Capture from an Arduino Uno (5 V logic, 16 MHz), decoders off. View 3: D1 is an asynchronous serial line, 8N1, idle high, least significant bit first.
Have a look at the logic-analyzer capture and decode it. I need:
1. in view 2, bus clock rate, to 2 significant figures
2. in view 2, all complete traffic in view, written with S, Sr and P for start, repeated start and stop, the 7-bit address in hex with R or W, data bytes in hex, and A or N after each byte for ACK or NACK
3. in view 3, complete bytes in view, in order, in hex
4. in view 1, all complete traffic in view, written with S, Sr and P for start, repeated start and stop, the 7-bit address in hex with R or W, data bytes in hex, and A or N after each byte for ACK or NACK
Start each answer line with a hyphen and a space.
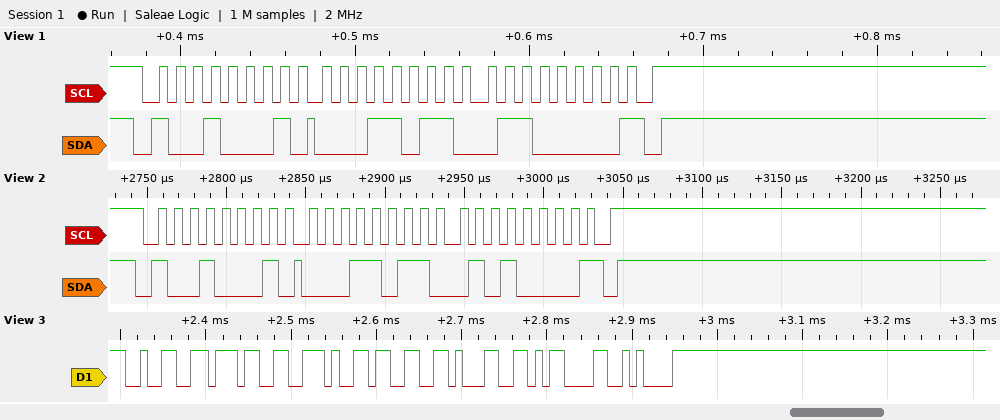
- 100 kHz
- S 48R A 1B A 50 N P
- 32 37 2E 33 31 0D 0A
- S 48R A 1B A 60 N P
